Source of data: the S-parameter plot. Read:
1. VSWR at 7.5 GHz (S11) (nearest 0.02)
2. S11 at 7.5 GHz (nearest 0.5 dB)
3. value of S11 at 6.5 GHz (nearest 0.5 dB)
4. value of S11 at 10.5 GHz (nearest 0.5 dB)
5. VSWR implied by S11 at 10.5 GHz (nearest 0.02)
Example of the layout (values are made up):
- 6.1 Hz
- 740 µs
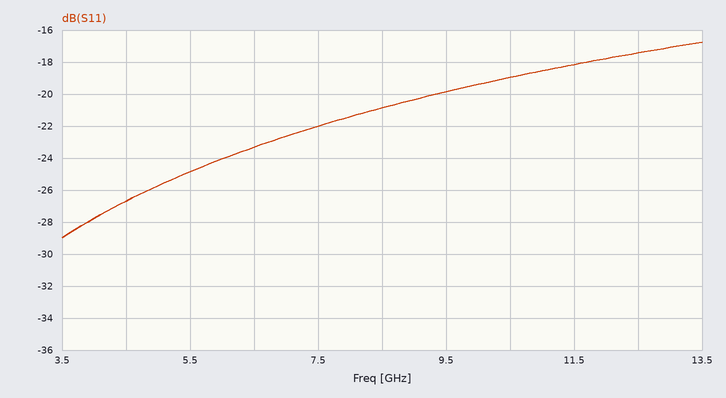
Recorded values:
- 1.18
- -22.0 dB
- -23.5 dB
- -19.0 dB
- 1.26
